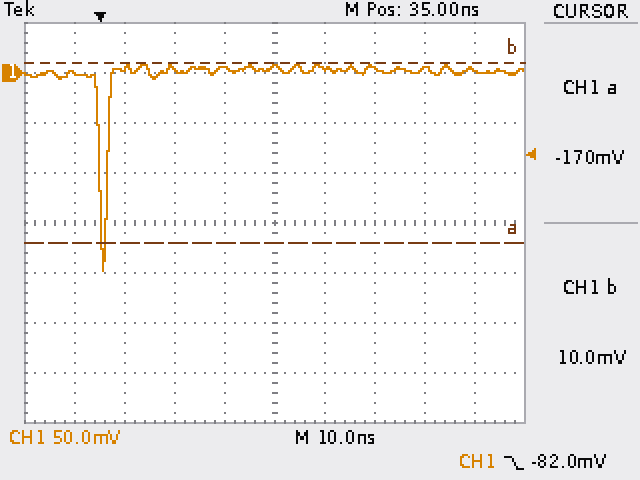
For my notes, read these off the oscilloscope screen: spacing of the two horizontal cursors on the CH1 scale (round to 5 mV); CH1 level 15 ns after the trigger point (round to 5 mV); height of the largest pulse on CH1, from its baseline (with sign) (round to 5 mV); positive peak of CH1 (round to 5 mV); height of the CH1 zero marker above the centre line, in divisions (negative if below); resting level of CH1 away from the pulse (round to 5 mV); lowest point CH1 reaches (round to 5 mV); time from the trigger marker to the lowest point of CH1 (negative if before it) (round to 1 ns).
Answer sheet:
180 mV
5 mV
-200 mV
10 mV
+3.0 div
0 mV
-200 mV
+1 ns
